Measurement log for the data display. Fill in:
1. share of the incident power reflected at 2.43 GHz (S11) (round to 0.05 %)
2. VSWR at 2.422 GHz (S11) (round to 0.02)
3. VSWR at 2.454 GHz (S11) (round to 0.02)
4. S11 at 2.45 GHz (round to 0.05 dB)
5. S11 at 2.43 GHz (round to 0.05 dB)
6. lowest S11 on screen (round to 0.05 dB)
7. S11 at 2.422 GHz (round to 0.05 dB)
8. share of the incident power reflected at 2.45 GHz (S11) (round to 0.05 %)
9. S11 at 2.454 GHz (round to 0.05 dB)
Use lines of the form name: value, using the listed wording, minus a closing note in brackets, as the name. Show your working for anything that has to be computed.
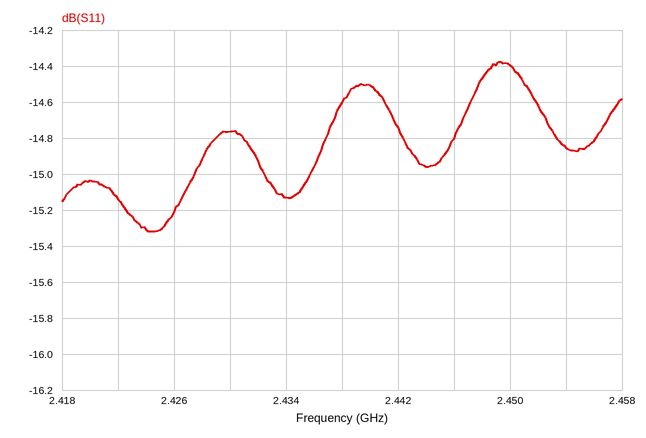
share of the incident power reflected at 2.43 GHz (S11): 10^(-14.75/10) ≈ 3.35 %
VSWR at 2.422 GHz (S11): |Γ| = 10^(-15.15/20) = 0.1748; VSWR = (1 + 0.1748)/(1 − 0.1748) ≈ 1.42
VSWR at 2.454 GHz (S11): |Γ| = 10^(-14.85/20) = 0.1809; VSWR = (1 + 0.1809)/(1 − 0.1809) ≈ 1.44
S11 at 2.45 GHz: -14.40 dB
S11 at 2.43 GHz: -14.75 dB
lowest S11 on screen: -15.30 dB
S11 at 2.422 GHz: -15.15 dB
share of the incident power reflected at 2.45 GHz (S11): 10^(-14.4/10) ≈ 3.63 %, so 3.65 % to the nearest 0.05 %
S11 at 2.454 GHz: -14.85 dB
